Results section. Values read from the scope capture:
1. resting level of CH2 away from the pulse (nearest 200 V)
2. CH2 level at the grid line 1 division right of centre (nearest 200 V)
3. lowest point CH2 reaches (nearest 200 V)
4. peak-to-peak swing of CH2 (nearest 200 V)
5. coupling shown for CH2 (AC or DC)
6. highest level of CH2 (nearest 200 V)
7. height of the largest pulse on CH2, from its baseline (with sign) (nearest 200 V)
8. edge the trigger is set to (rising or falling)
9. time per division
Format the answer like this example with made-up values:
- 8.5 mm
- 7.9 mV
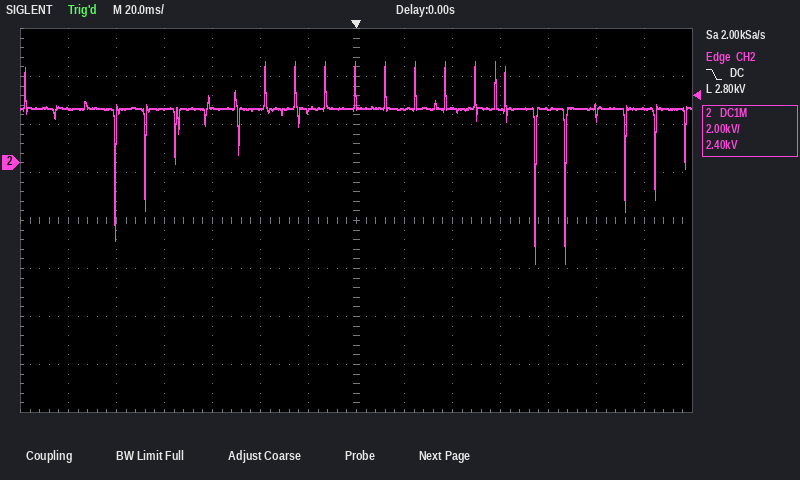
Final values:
- 2.2 kV
- 2.2 kV
- -4.2 kV
- 8.4 kV
- DC
- 4.2 kV
- -6.4 kV
- falling
- 20 ms
